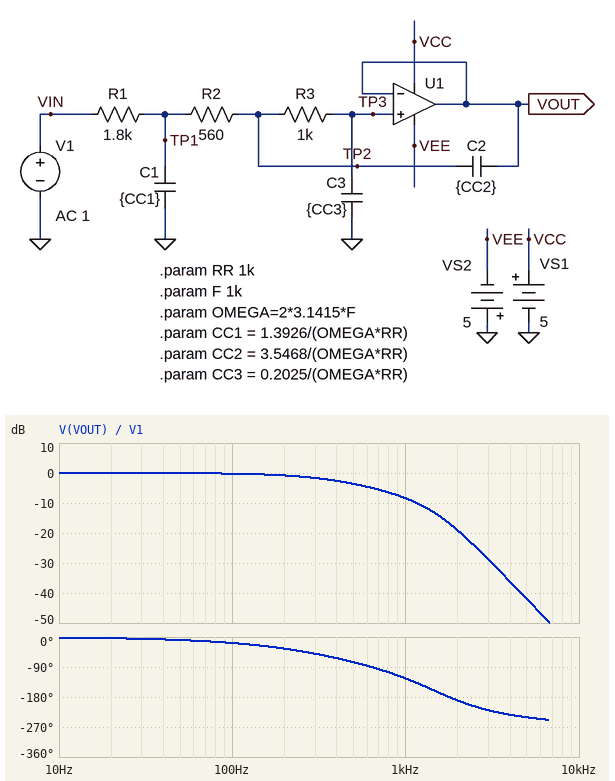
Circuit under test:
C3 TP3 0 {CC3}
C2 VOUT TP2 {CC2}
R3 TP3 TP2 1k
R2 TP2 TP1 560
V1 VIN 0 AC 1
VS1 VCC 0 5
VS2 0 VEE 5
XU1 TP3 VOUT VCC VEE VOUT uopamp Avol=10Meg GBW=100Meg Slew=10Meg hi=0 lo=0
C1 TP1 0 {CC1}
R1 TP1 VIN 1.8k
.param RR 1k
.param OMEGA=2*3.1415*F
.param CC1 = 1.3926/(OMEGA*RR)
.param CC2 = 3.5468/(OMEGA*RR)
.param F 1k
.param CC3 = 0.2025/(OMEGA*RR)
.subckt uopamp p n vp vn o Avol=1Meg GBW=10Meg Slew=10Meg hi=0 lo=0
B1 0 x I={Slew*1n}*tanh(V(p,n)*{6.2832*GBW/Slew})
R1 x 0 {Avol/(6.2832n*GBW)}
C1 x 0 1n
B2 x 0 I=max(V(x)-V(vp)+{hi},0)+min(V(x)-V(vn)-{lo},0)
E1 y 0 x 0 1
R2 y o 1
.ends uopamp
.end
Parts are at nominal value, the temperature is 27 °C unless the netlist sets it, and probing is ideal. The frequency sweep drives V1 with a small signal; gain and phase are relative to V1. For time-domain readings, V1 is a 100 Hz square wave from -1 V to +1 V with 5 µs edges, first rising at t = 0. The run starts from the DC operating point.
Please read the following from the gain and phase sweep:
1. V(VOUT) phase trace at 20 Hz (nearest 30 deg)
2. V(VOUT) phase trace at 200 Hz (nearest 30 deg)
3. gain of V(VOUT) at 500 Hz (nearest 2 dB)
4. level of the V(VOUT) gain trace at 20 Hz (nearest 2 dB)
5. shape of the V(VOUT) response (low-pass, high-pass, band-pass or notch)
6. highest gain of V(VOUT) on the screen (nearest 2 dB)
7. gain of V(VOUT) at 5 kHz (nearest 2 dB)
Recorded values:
0 deg
-30 deg
-4 dB
0 dB
low-pass
0 dB
-42 dB
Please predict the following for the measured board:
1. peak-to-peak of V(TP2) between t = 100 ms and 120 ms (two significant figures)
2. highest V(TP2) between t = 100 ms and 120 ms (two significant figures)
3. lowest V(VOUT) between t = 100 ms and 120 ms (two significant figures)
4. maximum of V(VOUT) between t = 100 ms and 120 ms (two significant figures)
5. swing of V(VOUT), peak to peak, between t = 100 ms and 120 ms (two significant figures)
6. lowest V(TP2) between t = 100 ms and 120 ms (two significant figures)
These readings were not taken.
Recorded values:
2.0 V
1.0 V
-1.0 V
1.0 V
2.0 V
-1.0 V
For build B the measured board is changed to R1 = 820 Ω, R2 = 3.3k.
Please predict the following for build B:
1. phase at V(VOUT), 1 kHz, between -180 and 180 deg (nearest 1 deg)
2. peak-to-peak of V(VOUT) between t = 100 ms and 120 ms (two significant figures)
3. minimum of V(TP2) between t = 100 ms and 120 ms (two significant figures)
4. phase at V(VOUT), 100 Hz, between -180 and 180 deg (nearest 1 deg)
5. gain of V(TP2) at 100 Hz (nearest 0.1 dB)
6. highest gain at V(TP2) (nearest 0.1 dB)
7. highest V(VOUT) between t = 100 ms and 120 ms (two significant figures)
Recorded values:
170 deg
3.0 V
-1.5 V
-13 deg
0.1 dB
2.5 dB
1.5 V
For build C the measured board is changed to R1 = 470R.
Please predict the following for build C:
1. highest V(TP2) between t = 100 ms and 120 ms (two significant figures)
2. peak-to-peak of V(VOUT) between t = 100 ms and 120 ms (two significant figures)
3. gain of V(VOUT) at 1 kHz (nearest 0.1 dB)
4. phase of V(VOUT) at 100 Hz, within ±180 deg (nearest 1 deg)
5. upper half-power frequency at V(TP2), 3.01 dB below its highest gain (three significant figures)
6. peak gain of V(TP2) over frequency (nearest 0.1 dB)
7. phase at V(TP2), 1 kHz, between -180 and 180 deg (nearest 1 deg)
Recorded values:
1.4 V
2.9 V
1.9 dB
-6 deg
1.40 kHz
2.1 dB
-75 deg
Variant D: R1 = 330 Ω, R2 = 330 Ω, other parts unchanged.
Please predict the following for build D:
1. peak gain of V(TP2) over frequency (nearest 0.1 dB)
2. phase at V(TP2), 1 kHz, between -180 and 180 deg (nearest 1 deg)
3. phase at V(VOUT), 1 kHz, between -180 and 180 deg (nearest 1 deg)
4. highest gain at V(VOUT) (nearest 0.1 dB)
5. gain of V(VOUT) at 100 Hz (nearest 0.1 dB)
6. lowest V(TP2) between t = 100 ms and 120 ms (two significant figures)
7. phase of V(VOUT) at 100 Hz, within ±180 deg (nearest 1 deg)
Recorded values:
2.4 dB
-48 deg
-60 deg
2.2 dB
0 dB
-1.5 V
-5 deg
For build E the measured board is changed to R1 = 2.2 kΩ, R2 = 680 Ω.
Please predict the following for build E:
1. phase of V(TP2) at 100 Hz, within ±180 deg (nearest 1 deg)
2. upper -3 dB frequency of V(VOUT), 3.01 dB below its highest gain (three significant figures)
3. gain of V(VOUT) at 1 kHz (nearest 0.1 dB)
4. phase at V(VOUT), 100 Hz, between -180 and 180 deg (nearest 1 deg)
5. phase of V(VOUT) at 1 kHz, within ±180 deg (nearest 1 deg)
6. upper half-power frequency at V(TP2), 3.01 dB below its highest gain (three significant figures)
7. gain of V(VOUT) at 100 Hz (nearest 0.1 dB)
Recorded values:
-20 deg
345 Hz
-10.0 dB
-22 deg
-132 deg
347 Hz
-0.4 dB
